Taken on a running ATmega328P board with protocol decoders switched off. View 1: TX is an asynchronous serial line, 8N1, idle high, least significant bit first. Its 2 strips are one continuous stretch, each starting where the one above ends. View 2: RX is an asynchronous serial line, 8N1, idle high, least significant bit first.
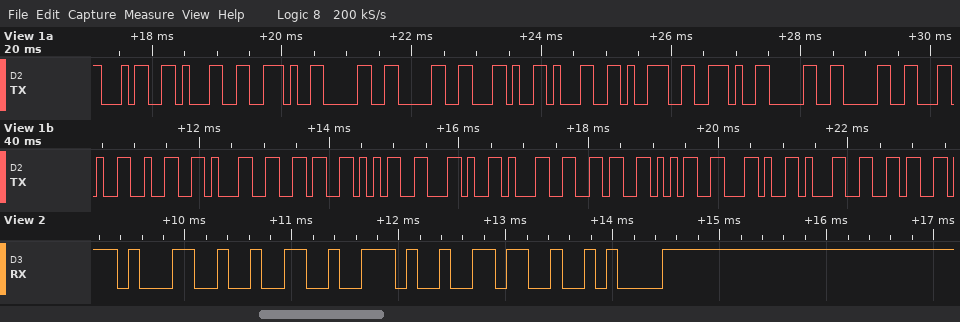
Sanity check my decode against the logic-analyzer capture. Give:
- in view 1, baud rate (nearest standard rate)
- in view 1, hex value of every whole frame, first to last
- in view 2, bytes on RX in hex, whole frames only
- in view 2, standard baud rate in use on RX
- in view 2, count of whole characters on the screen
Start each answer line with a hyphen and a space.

- 9600 baud
- 34 31 2E 30 30 2C 31 39 2E 30 30 2C 32 31 36 35 2C 31 36 35 2C 31 36
- 31 32 2E 36 0A
- 9600 baud
- 5
